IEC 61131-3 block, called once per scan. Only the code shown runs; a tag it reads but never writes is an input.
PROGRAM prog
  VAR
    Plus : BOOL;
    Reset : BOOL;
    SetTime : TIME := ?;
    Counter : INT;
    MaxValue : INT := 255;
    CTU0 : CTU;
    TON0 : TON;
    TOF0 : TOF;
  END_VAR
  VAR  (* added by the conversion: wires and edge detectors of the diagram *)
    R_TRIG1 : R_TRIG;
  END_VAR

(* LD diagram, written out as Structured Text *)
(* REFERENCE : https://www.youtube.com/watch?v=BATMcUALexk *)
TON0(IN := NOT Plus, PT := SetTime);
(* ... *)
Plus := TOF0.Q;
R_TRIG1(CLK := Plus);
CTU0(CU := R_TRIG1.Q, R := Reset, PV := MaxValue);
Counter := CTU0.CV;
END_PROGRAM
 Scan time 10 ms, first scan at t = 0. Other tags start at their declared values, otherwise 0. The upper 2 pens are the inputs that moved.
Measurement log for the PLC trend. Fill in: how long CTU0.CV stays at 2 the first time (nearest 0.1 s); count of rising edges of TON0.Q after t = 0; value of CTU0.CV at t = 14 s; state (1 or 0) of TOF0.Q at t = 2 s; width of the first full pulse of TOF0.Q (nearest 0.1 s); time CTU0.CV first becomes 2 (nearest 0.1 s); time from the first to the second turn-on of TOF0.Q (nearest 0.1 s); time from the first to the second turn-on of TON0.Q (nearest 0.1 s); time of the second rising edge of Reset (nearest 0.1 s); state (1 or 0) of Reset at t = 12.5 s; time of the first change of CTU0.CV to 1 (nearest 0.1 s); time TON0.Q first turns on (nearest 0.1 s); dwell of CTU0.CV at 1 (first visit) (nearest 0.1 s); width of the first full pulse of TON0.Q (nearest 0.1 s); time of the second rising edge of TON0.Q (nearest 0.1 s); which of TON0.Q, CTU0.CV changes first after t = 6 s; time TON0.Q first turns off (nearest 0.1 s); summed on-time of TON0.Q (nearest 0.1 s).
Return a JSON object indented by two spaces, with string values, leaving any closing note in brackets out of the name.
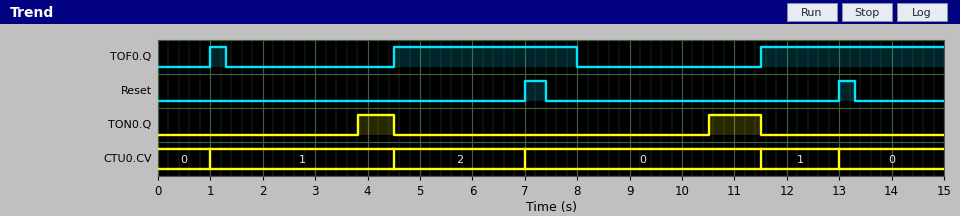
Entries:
{
  "how long CTU0.CV stays at 2 the first time": "2.5 s",
  "count of rising edges of TON0.Q after t = 0": "2",
  "value of CTU0.CV at t = 14 s": "0",
  "state (1 or 0) of TOF0.Q at t = 2 s": "0",
  "width of the first full pulse of TOF0.Q": "0.3 s",
  "time CTU0.CV first becomes 2": "4.5 s",
  "time from the first to the second turn-on of TOF0.Q": "3.5 s",
  "time from the first to the second turn-on of TON0.Q": "6.7 s",
  "time of the second rising edge of Reset": "13.0 s",
  "state (1 or 0) of Reset at t = 12.5 s": "0",
  "time of the first change of CTU0.CV to 1": "1.0 s",
  "time TON0.Q first turns on": "3.8 s",
  "dwell of CTU0.CV at 1 (first visit)": "3.5 s",
  "width of the first full pulse of TON0.Q": "0.7 s",
  "time of the second rising edge of TON0.Q": "10.5 s",
  "which of TON0.Q, CTU0.CV changes first after t = 6 s": "CTU0.CV",
  "time TON0.Q first turns off": "4.5 s",
  "summed on-time of TON0.Q": "1.7 s"
}
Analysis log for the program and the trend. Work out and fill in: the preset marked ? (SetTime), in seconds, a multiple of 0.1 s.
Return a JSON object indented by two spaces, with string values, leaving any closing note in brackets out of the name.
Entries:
{
  "the preset marked ? (SetTime), in seconds, a multiple of 0.1 s": "2.5 s"
}
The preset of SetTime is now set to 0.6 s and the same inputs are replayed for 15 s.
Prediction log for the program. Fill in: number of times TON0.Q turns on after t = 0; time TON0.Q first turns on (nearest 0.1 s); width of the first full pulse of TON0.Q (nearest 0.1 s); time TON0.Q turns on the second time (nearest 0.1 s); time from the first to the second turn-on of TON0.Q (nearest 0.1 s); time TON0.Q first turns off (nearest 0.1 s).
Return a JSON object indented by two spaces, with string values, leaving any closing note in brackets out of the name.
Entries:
{
  "number of times TON0.Q turns on after t = 0": "3",
  "time TON0.Q first turns on": "0.6 s",
  "width of the first full pulse of TON0.Q": "0.4 s",
  "time TON0.Q turns on the second time": "1.9 s",
  "time from the first to the second turn-on of TON0.Q": "1.3 s",
  "time TON0.Q first turns off": "1.0 s"
}
